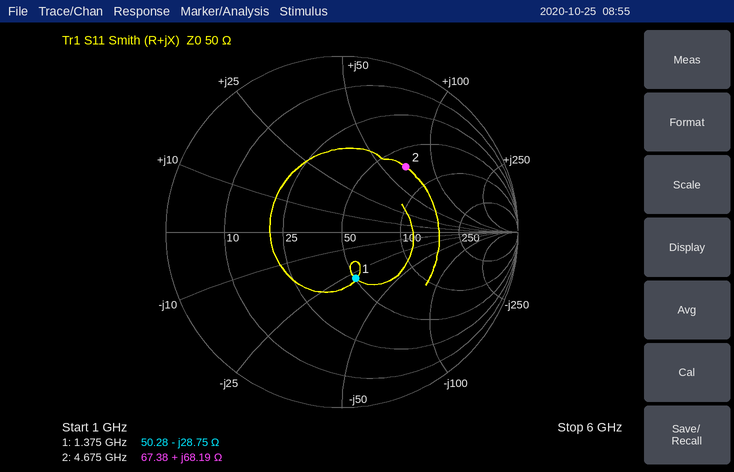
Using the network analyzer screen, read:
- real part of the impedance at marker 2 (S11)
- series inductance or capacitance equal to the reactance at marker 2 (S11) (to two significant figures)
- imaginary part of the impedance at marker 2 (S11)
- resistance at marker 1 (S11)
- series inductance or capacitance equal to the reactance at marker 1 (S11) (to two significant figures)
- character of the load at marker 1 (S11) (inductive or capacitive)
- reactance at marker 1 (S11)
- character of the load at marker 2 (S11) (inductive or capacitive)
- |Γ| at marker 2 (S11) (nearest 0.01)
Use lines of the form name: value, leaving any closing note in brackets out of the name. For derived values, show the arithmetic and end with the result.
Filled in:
real part of the impedance at marker 2: 67.38 Ω
series inductance or capacitance equal to the reactance at marker 2 (S11): L = 68.19 Ω/(2π × 4.675 GHz) ≈ 2.3 nH
imaginary part of the impedance at marker 2: +68.19 Ω
resistance at marker 1: 50.28 Ω
series inductance or capacitance equal to the reactance at marker 1 (S11): C = 1/(2π × 1.375 GHz × 28.75 Ω) ≈ 4.0 pF
character of the load at marker 1 (S11): capacitive
reactance at marker 1: -28.75 Ω
character of the load at marker 2 (S11): inductive
|Γ| at marker 2 (S11): 0.52
